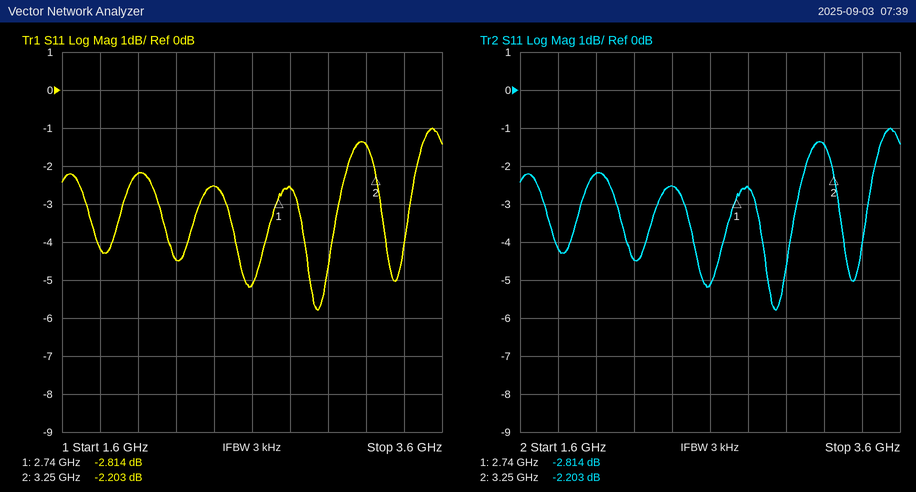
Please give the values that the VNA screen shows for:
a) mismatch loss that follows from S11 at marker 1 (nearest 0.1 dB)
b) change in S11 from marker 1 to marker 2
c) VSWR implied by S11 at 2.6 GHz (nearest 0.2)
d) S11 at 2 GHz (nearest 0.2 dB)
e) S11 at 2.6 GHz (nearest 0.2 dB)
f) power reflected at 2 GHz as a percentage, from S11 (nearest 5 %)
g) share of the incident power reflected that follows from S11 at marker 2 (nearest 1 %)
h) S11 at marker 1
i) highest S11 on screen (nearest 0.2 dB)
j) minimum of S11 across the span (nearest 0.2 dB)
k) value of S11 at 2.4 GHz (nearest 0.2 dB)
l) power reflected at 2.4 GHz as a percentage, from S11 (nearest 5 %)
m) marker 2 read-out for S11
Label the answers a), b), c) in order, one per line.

a) 3.2 dB
b) 0.611 dB
c) 3.4
d) -2.2 dB
e) -5.2 dB
f) 60 %
g) 60 %
h) -2.814 dB
i) -1.0 dB
j) -5.8 dB
k) -2.6 dB
l) 55 %
m) -2.203 dB
